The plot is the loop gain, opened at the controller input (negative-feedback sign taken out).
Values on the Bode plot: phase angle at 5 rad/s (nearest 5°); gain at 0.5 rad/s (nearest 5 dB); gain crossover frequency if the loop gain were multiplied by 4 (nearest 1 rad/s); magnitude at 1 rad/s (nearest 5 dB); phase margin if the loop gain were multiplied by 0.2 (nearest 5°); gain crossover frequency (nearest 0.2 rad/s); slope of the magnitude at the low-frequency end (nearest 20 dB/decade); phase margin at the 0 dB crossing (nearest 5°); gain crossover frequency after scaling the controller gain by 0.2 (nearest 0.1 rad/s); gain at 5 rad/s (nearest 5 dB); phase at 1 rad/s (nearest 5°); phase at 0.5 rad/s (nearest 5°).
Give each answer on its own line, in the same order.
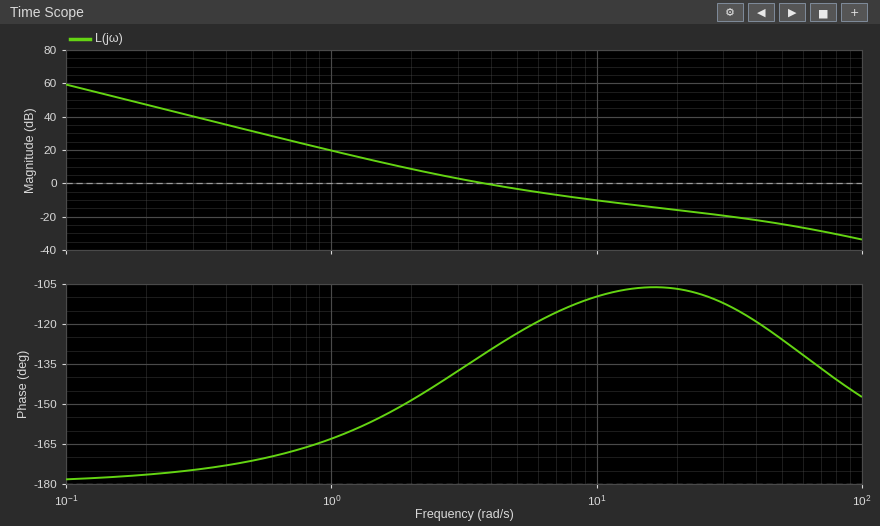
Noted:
-125°
30 dB
12 rad/s
20 dB
25°
3.8 rad/s
-40 dB/decade
50°
1.4 rad/s
-5 dB
-165°
-170°
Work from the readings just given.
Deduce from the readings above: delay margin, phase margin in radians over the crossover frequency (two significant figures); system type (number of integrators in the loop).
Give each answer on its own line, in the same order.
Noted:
0.23 s
2
